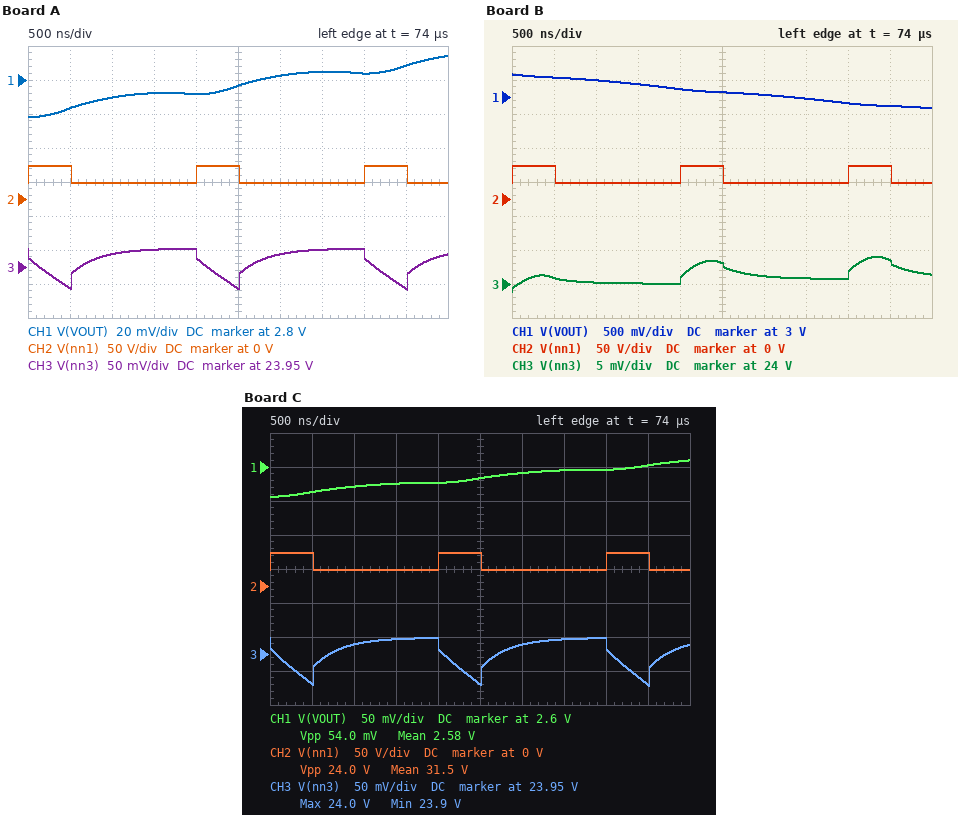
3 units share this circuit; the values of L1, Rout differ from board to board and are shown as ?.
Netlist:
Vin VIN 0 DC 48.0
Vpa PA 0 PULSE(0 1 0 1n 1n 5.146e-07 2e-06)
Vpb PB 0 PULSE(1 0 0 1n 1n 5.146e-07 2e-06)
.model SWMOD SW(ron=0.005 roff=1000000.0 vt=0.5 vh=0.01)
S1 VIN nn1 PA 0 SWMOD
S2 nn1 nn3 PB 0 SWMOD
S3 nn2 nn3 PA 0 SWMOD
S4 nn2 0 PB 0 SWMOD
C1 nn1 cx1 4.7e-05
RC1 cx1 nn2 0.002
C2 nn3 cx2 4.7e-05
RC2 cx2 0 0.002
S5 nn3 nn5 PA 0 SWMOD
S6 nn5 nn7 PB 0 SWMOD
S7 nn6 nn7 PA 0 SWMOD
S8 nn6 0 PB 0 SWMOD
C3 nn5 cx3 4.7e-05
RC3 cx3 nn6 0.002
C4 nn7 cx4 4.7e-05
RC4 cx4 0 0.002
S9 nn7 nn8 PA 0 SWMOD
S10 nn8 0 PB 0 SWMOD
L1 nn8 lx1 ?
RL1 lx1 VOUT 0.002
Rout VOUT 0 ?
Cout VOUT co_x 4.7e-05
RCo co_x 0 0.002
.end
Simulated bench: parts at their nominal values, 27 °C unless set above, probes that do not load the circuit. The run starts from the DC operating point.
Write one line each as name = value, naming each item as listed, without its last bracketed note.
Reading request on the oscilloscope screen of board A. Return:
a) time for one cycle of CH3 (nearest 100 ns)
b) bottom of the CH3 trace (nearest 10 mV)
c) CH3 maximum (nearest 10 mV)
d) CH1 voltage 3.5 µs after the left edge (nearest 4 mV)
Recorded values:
time for one cycle of CH3 = 2.0 µs
bottom of the CH3 trace = 23.92 V
CH3 maximum = 23.98 V
CH1 voltage 3.5 µs after the left edge = 2.804 V
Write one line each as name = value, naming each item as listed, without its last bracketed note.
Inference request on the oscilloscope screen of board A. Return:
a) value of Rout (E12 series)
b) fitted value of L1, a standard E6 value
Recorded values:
value of Rout = 0.15 Ω
fitted value of L1, a standard E6 value = 4.7 µH
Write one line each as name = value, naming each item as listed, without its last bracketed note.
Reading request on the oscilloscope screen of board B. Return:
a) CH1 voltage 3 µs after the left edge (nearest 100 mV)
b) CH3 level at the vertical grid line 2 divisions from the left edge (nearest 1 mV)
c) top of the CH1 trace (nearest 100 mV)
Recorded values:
CH1 voltage 3 µs after the left edge = 3.0 V
CH3 level at the vertical grid line 2 divisions from the left edge = 24.000 V
top of the CH1 trace = 3.3 V
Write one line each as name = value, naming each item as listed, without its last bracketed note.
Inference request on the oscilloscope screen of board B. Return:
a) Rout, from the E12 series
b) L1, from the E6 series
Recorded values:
Rout, from the E12 series = 0.82 Ω
L1, from the E6 series = 1 µH
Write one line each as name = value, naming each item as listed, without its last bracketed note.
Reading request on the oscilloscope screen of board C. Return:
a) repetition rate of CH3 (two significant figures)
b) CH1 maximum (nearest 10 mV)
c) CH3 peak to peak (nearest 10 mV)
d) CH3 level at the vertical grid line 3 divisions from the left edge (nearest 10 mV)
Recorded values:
repetition rate of CH3 = 500 kHz
CH1 maximum = 2.61 V
CH3 peak to peak = 70 mV
CH3 level at the vertical grid line 3 divisions from the left edge = 23.97 V
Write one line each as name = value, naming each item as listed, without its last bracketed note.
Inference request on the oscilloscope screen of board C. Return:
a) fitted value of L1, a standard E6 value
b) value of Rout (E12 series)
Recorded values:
fitted value of L1, a standard E6 value = 4.7 µH
value of Rout = 0.12 Ω
